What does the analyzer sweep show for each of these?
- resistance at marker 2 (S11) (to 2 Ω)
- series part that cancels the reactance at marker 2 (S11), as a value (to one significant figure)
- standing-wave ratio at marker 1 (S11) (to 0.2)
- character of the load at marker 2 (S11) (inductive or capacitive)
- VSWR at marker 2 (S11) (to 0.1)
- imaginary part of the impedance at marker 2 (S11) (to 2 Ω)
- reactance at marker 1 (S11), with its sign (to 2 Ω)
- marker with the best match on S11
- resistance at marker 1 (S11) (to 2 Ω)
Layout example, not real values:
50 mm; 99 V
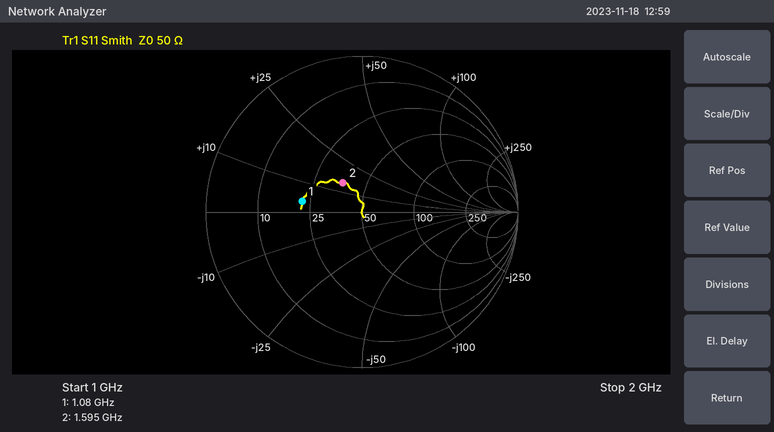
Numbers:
36 Ω; 7 pF; 2.2; inductive; 1.6; +14 Ω; +4 Ω; marker 2; 22 Ω
